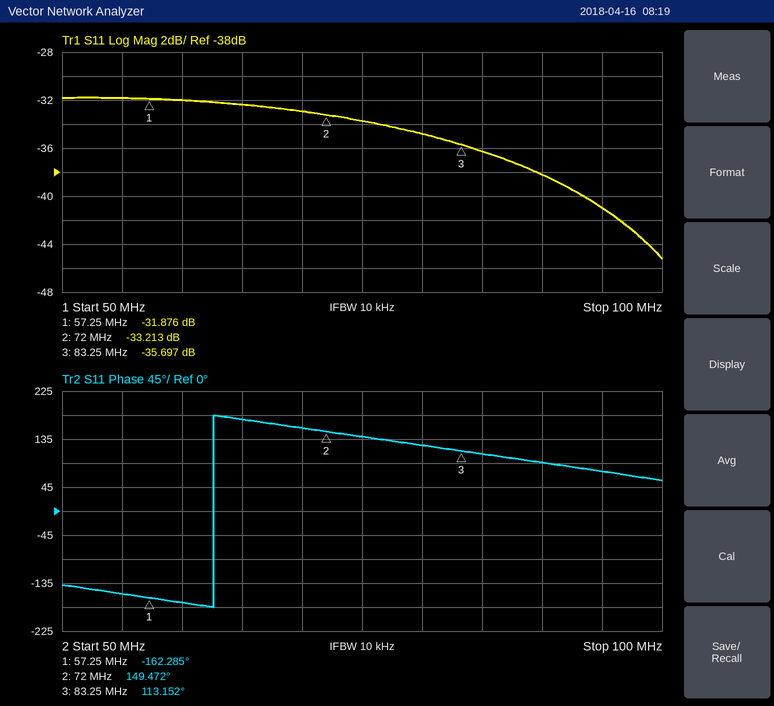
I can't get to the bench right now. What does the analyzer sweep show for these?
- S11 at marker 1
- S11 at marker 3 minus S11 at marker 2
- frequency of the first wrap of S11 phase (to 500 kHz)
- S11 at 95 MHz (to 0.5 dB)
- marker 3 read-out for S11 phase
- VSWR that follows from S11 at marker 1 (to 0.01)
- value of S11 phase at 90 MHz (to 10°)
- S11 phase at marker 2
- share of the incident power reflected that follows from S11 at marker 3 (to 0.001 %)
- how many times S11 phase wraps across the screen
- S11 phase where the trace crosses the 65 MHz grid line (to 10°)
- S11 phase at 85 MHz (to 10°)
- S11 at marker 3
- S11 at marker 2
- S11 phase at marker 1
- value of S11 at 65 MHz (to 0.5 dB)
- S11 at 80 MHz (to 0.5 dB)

-31.876 dB
-2.484 dB
62.5 MHz
-41.0 dB
113.152°
1.05
90°
149.472°
0.027 %
1
170°
110°
-35.697 dB
-33.213 dB
-162.285°
-32.5 dB
-35.0 dB
